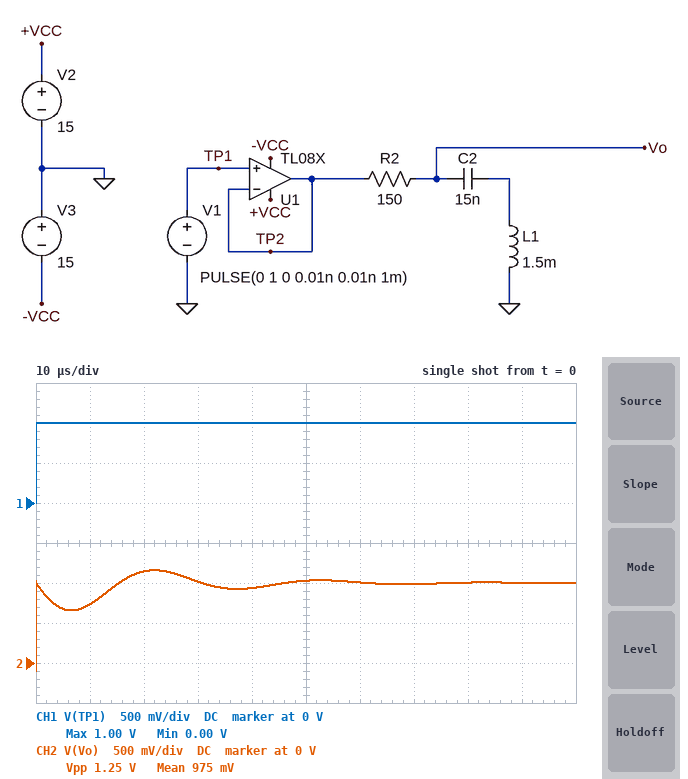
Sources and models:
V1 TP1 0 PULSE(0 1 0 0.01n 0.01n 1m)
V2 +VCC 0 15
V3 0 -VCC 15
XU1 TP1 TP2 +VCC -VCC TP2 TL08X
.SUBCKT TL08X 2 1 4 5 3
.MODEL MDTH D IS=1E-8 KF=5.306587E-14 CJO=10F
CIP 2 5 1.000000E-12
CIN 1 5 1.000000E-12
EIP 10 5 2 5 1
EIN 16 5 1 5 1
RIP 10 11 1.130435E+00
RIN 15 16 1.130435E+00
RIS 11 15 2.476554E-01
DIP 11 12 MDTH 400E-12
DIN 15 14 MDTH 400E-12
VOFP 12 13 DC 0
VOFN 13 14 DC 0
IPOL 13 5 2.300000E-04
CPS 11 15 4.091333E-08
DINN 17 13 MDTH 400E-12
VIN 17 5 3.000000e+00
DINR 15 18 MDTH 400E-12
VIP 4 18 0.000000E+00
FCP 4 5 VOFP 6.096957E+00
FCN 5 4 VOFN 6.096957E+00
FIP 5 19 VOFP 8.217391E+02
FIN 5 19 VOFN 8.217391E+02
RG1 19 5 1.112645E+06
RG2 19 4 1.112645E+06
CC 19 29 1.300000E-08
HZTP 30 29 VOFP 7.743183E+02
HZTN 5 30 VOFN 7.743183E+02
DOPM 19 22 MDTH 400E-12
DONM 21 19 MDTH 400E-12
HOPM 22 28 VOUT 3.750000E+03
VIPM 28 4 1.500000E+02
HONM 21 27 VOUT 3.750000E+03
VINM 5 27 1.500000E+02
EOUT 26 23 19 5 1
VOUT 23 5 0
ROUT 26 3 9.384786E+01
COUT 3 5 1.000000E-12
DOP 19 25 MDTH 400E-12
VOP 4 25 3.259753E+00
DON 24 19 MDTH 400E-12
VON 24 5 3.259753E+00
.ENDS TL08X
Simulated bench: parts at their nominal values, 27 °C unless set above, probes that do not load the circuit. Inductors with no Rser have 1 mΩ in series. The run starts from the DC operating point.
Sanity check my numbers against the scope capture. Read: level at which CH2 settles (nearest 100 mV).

1.0 V
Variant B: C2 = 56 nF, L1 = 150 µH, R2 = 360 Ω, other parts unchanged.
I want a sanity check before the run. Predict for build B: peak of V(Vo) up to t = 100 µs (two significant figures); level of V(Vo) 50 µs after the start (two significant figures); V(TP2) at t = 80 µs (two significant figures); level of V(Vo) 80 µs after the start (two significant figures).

990 mV
920 mV
1.0 V
980 mV
